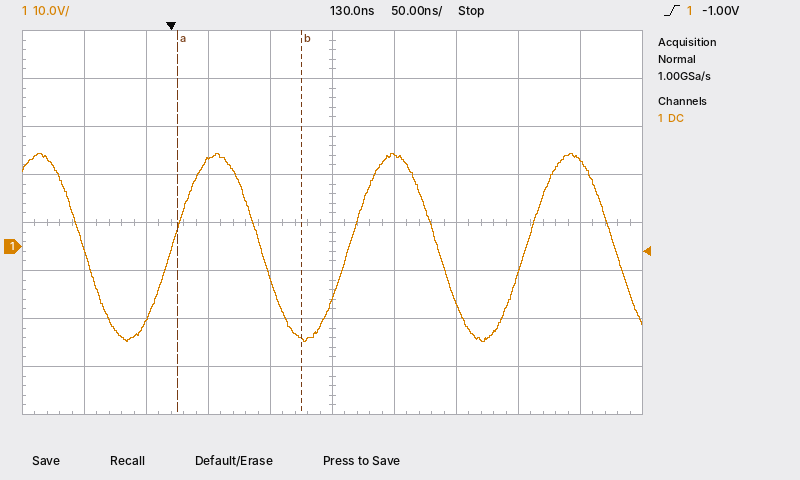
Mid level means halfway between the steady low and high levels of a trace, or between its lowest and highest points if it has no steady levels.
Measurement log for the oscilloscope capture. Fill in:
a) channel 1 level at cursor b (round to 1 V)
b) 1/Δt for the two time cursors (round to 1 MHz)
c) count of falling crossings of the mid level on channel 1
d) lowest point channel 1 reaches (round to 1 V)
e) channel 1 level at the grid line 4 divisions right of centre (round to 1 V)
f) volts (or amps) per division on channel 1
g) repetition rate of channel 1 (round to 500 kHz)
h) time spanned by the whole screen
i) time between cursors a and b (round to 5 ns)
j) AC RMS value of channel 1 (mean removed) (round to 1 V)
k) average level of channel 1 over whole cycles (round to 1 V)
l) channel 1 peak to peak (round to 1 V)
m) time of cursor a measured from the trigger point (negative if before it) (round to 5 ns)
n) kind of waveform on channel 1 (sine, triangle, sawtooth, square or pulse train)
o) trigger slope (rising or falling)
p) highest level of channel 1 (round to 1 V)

-19 V
10 MHz
4
-20 V
18 V
10 V
7.0 MHz
500 ns
100 ns
14 V
0 V
39 V
+5 ns
sine
rising
19 V
